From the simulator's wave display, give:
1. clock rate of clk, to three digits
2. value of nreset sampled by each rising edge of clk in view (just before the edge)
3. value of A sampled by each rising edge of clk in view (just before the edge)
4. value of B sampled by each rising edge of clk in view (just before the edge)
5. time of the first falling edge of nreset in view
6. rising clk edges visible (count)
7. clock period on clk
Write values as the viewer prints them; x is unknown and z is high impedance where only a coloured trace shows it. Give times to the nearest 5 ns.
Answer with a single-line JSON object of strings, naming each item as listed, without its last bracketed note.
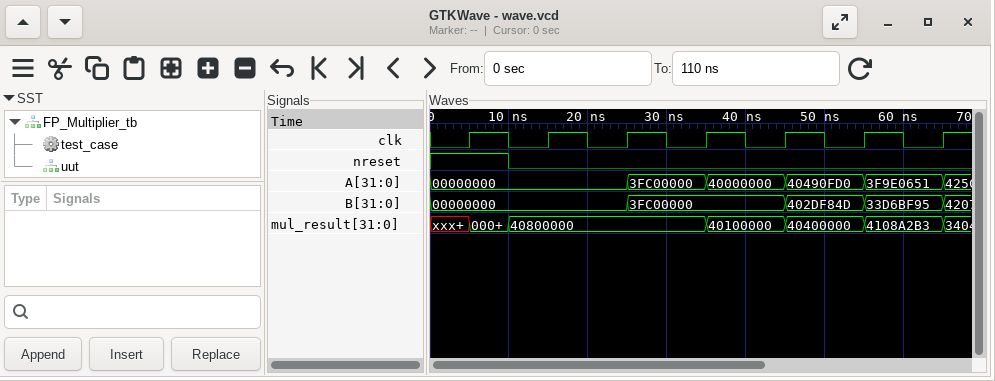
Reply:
{"clock rate of clk, to three digits": "100 MHz", "value of nreset sampled by each rising edge of clk in view": "1 0 0 0 0 0 0", "value of A sampled by each rising edge of clk in view": "00000000, 00000000, 00000000, 3FC00000, 40000000, 40490FD0, 3F9E0651", "value of B sampled by each rising edge of clk in view": "00000000, 00000000, 00000000, 3FC00000, 3FC00000, 402DF84D, 33D6BF95", "time of the first falling edge of nreset in view": "10 ns", "rising clk edges visible": "7", "clock period on clk": "10 ns"}
